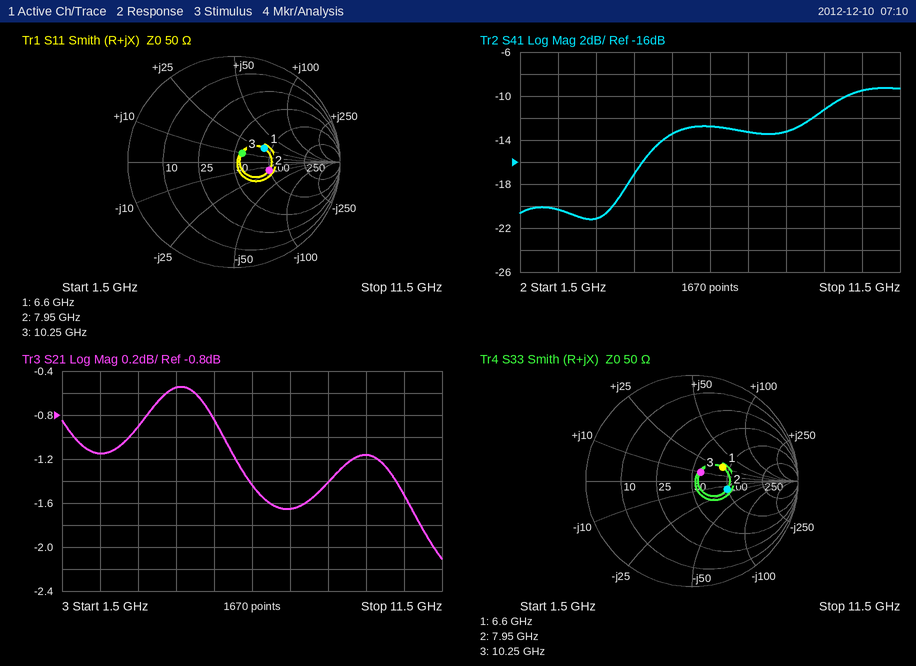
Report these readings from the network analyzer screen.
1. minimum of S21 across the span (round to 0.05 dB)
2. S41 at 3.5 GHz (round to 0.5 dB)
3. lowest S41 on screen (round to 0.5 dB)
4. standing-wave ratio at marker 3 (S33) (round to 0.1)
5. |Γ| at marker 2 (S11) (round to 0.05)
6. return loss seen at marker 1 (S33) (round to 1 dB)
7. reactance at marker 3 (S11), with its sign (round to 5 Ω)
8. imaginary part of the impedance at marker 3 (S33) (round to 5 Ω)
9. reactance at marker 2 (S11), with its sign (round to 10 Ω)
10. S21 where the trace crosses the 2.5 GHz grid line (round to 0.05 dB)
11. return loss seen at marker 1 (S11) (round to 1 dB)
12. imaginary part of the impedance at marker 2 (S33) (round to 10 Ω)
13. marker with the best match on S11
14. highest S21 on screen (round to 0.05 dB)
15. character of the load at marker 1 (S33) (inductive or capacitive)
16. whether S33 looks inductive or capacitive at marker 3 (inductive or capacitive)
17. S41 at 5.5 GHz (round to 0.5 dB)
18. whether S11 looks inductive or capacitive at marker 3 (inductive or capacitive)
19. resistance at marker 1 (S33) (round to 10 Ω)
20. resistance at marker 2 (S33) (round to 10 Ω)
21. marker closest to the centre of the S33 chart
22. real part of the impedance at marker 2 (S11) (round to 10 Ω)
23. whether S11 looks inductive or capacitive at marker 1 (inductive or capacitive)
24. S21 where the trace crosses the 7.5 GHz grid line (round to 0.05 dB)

-2.10 dB
-21.0 dB
-21.0 dB
1.3
0.35
10 dB
+10 Ω
+10 Ω
-20 Ω
-1.15 dB
10 dB
-20 Ω
marker 3
-0.55 dB
inductive
inductive
-13.5 dB
inductive
90 Ω
100 Ω
marker 3
100 Ω
inductive
-1.65 dB
